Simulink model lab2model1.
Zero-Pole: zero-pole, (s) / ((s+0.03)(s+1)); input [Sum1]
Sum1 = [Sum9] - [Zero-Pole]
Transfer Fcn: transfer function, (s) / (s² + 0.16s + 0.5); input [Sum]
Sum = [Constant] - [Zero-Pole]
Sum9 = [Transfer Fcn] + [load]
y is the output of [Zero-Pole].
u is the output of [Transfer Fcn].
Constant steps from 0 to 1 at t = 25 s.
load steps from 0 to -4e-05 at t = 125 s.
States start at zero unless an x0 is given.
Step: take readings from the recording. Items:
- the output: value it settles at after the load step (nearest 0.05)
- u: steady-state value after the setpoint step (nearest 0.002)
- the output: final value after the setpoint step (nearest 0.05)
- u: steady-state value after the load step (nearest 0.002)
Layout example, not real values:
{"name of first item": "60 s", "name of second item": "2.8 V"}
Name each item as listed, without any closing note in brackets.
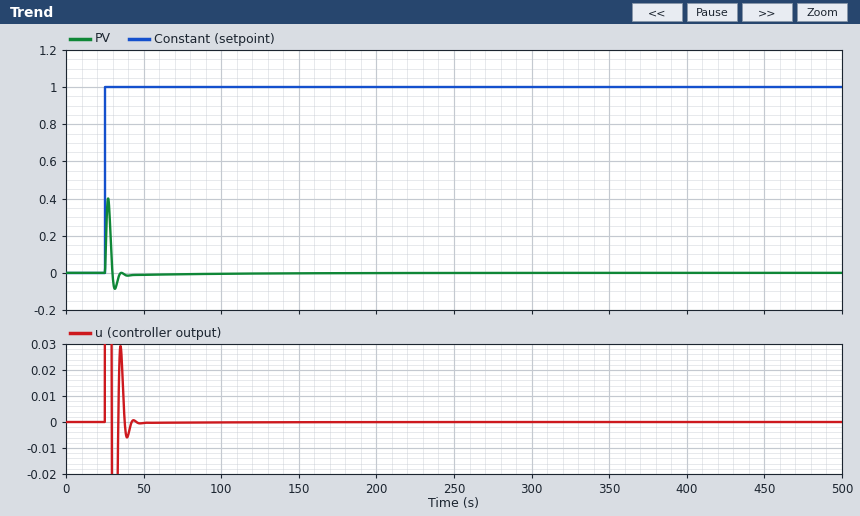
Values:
{"the output: value it settles at after the load step": "0.00", "u: steady-state value after the setpoint step": "0.000", "the output: final value after the setpoint step": "0.00", "u: steady-state value after the load step": "0.000"}
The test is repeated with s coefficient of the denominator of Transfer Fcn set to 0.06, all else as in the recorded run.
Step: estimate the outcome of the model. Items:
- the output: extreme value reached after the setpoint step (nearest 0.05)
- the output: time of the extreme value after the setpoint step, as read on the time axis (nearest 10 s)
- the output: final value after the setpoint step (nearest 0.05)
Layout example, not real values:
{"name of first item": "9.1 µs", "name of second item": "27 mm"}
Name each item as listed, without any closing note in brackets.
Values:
{"the output: extreme value reached after the setpoint step": "0.45", "the output: time of the extreme value after the setpoint step, as read on the time axis": "30 s", "the output: final value after the setpoint step": "0.00"}
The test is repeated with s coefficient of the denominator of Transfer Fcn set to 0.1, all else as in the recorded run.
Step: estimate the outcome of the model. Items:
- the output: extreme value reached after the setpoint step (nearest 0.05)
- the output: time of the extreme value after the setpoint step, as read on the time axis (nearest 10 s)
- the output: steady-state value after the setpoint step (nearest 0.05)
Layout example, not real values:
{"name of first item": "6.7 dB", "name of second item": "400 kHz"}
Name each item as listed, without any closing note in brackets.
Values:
{"the output: extreme value reached after the setpoint step": "0.40", "the output: time of the extreme value after the setpoint step, as read on the time axis": "30 s", "the output: steady-state value after the setpoint step": "0.00"}
